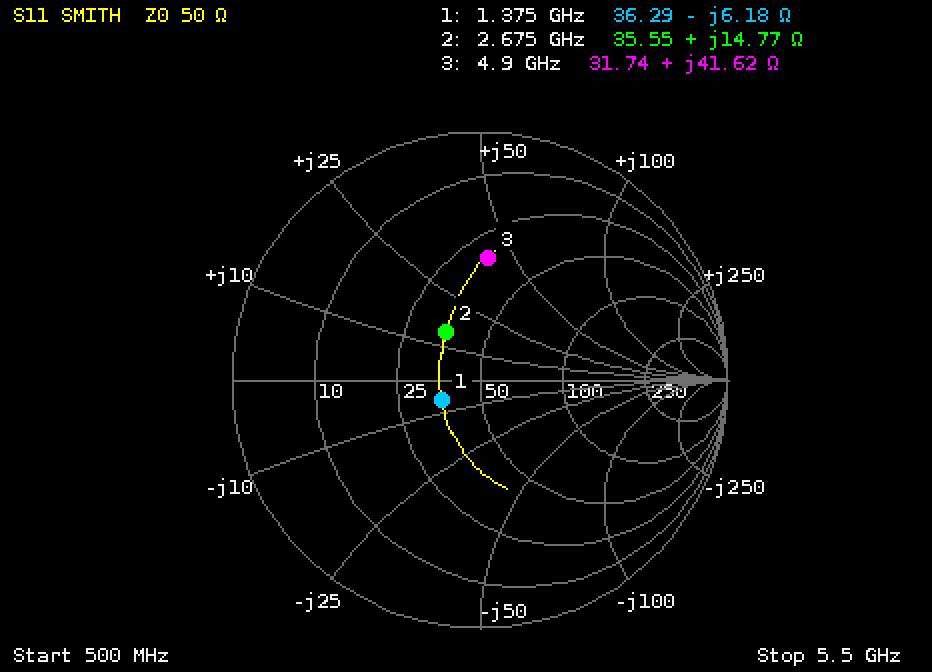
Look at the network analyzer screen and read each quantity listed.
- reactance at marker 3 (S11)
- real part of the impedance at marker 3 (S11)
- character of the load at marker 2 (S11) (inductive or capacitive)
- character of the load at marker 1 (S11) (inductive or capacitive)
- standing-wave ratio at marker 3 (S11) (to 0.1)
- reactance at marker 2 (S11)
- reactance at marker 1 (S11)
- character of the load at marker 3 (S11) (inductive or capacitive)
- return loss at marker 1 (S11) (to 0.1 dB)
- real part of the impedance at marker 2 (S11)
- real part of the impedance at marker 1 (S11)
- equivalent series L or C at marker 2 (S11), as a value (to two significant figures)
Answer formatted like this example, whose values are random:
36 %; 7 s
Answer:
+41.62 Ω; 31.74 Ω; inductive; capacitive; 3.0; +14.77 Ω; -6.18 Ω; inductive; 15.2 dB; 35.55 Ω; 36.29 Ω; 880 pH
